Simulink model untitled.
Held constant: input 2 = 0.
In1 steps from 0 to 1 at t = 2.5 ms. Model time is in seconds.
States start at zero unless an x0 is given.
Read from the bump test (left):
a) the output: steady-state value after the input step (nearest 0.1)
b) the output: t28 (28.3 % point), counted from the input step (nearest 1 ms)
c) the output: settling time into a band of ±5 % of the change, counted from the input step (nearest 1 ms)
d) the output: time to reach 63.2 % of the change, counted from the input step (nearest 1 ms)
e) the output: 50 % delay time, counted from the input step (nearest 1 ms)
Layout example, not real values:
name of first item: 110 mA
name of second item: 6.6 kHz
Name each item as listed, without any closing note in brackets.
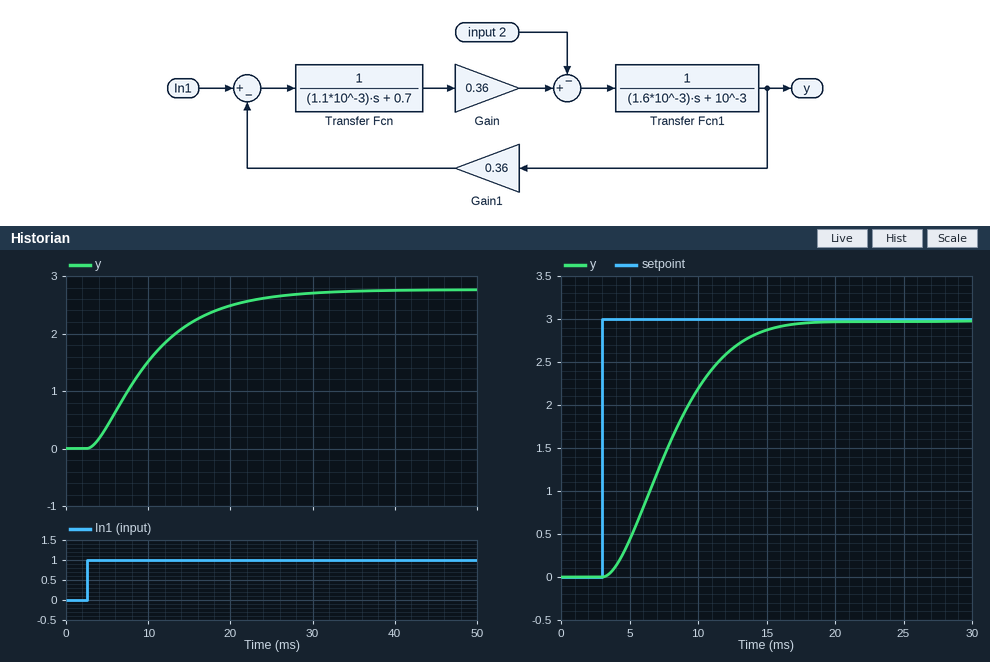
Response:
the output: steady-state value after the input step: 2.8
the output: t28 (28.3 % point), counted from the input step: 4 ms
the output: settling time into a band of ±5 % of the change, counted from the input step: 22 ms
the output: time to reach 63.2 % of the change, counted from the input step: 9 ms
the output: 50 % delay time, counted from the input step: 7 ms
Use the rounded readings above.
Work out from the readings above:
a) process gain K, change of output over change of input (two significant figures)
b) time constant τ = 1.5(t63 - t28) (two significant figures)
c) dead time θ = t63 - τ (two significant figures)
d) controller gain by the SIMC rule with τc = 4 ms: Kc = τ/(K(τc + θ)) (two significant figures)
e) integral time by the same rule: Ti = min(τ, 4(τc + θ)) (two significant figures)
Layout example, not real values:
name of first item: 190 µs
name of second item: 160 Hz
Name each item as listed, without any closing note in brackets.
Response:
process gain K, change of output over change of input: 2.8
time constant τ = 1.5(t63 - t28): 7.5 ms
dead time θ = t63 - τ: 1.5 ms
controller gain by the SIMC rule with τc = 4 ms: Kc = τ/(K(τc + θ)): 0.49
integral time by the same rule: Ti = min(τ, 4(τc + θ)): 7.5 ms
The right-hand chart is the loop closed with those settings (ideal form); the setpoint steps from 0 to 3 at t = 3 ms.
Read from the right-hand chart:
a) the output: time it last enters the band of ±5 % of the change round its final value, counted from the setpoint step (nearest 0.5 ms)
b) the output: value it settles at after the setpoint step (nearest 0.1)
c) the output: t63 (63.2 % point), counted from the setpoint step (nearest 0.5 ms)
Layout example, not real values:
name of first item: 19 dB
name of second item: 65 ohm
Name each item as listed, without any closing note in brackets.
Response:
the output: time it last enters the band of ±5 % of the change round its final value, counted from the setpoint step: 11.5 ms
the output: value it settles at after the setpoint step: 3.0
the output: t63 (63.2 % point), counted from the setpoint step: 6.0 ms
